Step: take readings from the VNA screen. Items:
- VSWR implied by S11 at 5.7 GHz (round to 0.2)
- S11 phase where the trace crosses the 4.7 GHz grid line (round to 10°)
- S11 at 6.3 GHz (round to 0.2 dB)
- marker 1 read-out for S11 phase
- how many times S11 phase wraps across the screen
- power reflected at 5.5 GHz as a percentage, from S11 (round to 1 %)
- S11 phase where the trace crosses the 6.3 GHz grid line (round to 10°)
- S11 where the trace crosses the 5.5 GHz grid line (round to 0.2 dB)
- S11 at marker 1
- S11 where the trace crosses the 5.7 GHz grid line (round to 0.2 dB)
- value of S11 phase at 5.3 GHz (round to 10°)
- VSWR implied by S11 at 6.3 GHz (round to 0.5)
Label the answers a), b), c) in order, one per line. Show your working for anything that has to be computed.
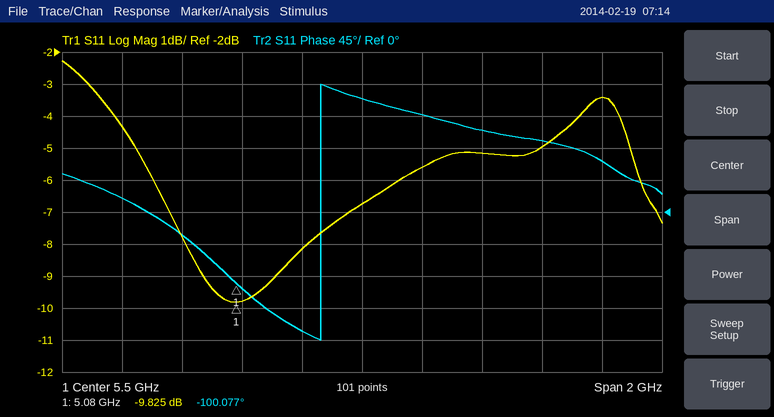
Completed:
a) |Γ| = 10^(-5.6/20) = 0.5248; VSWR = (1 + 0.5248)/(1 − 0.5248) ≈ 3.2
b) 20°
c) -3.4 dB
d) -100.077°
e) 1
f) 10^(-6.8/10) ≈ 21 %
g) 70°
h) -6.8 dB
i) -9.825 dB
j) -5.6 dB
k) -170°
l) |Γ| = 10^(-3.4/20) = 0.6761; VSWR = (1 + 0.6761)/(1 − 0.6761) ≈ 5.17, so 5.0 to the nearest 0.5
